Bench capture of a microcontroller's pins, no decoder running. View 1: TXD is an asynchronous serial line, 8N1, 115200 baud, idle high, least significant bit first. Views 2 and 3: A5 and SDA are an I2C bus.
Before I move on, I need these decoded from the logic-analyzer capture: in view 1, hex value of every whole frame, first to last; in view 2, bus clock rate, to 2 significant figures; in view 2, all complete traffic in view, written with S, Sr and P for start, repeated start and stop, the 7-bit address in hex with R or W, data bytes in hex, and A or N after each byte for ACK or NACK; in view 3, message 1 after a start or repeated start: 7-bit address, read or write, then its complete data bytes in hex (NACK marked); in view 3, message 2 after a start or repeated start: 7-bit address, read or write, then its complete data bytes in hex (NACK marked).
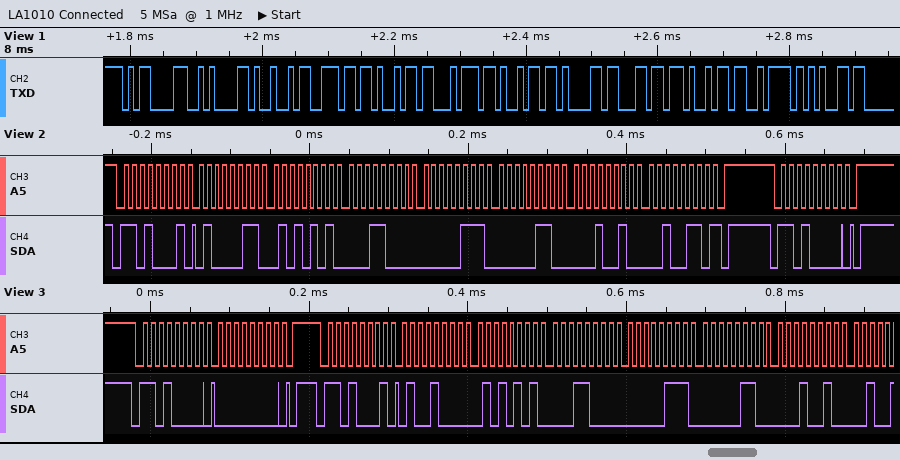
0x0D 0x0A 0x49 0x6E 0x69 0x74 0x69 0x61 0x6C 0x69 0x7A 0x65
100 kHz
S 68R A 43 A 55 A 18 A 07 A 06 A 12 A 26 N P S 68W A P
0x68 write: 00
0x68 read: 48 55 18 07 06 12
